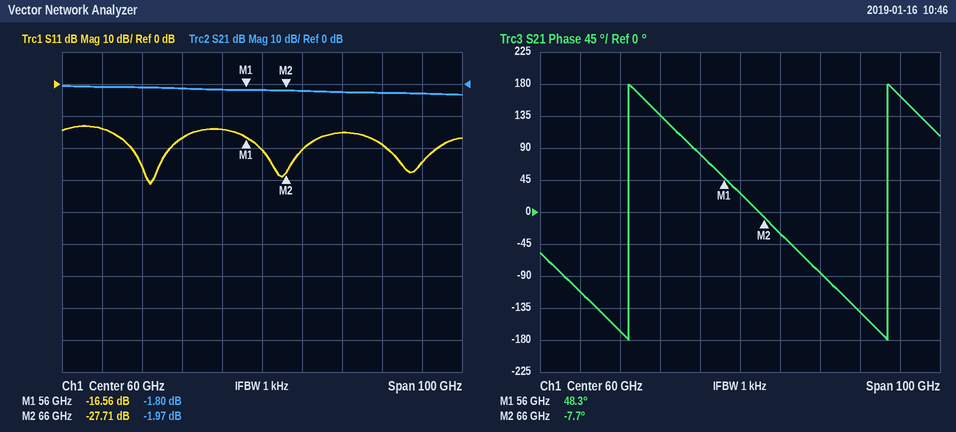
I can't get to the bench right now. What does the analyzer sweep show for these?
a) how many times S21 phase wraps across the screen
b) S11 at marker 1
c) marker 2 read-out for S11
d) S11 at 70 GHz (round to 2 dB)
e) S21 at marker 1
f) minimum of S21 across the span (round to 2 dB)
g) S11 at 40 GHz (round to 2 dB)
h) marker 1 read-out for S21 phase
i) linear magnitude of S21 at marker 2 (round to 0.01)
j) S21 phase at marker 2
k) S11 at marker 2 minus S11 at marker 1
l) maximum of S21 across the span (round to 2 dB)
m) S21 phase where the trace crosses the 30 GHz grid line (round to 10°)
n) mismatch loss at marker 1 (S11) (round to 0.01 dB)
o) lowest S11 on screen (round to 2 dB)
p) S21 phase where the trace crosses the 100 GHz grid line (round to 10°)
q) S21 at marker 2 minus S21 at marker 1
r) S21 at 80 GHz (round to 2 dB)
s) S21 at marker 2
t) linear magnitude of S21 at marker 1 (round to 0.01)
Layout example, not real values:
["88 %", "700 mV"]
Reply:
["2", "-16.56 dB", "-27.71 dB", "-20 dB", "-1.80 dB", "-4 dB", "-16 dB", "48.3°", "0.80", "-7.7°", "-11.15 dB", "0 dB", "-170°", "0.10 dB", "-32 dB", "160°", "-0.17 dB", "-2 dB", "-1.97 dB", "0.81"]
